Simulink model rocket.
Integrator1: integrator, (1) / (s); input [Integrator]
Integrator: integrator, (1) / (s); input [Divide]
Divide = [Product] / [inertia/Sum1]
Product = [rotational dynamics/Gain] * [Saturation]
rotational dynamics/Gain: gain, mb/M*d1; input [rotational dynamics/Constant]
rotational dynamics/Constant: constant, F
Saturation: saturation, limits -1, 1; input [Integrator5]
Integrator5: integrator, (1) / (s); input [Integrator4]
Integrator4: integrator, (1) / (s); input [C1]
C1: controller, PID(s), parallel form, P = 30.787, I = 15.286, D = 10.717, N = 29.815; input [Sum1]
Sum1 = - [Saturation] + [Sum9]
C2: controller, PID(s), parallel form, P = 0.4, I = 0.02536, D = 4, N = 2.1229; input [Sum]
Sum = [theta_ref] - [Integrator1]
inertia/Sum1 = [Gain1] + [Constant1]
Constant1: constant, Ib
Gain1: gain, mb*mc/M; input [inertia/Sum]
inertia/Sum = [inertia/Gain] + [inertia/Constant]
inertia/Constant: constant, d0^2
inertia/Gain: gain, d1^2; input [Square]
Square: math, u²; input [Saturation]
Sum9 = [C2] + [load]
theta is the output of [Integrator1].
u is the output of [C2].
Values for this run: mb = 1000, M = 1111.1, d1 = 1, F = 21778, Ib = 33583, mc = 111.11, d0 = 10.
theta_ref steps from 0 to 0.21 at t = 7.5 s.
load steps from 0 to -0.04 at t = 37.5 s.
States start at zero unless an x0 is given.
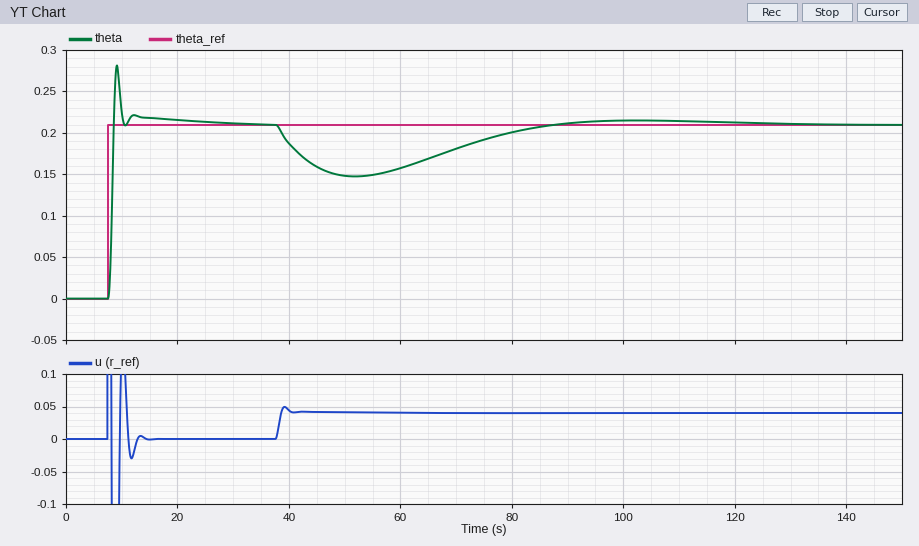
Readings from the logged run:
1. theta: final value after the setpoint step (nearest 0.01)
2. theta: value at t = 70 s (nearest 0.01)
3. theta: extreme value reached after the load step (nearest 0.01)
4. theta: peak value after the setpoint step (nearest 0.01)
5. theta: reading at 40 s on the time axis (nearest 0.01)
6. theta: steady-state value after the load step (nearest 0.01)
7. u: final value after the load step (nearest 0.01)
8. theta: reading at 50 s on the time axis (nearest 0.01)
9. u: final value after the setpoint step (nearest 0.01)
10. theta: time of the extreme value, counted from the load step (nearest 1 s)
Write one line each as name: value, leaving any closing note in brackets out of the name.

theta: final value after the setpoint step: 0.21
theta: value at t = 70 s: 0.18
theta: extreme value reached after the load step: 0.15
theta: peak value after the setpoint step: 0.28
theta: reading at 40 s on the time axis: 0.19
theta: steady-state value after the load step: 0.21
u: final value after the load step: 0.04
theta: reading at 50 s on the time axis: 0.15
u: final value after the setpoint step: 0.00
theta: time of the extreme value, counted from the load step: 14 s
